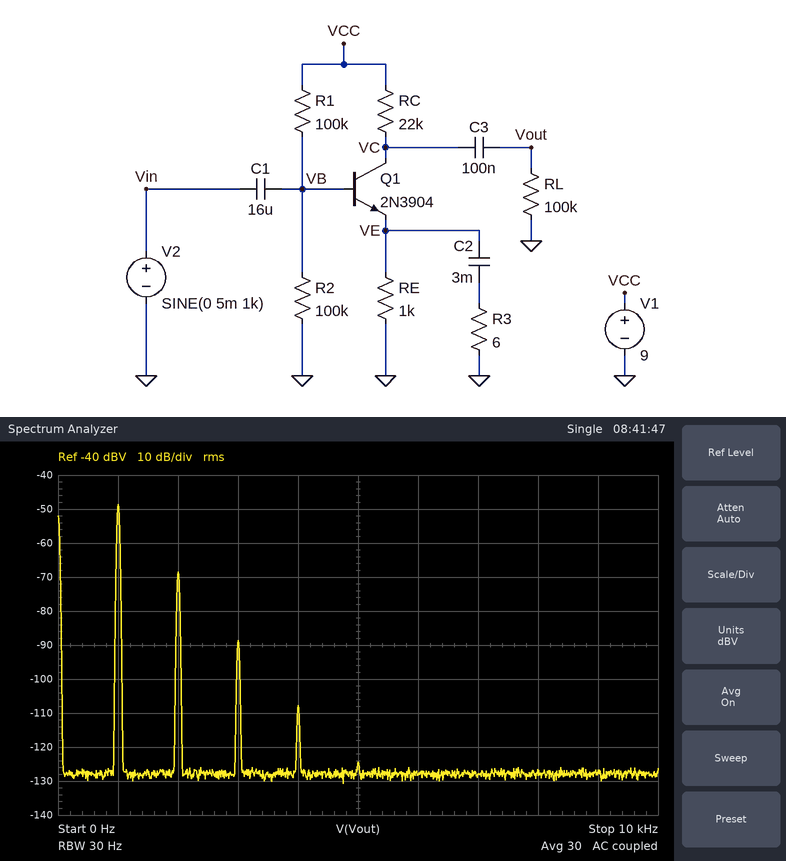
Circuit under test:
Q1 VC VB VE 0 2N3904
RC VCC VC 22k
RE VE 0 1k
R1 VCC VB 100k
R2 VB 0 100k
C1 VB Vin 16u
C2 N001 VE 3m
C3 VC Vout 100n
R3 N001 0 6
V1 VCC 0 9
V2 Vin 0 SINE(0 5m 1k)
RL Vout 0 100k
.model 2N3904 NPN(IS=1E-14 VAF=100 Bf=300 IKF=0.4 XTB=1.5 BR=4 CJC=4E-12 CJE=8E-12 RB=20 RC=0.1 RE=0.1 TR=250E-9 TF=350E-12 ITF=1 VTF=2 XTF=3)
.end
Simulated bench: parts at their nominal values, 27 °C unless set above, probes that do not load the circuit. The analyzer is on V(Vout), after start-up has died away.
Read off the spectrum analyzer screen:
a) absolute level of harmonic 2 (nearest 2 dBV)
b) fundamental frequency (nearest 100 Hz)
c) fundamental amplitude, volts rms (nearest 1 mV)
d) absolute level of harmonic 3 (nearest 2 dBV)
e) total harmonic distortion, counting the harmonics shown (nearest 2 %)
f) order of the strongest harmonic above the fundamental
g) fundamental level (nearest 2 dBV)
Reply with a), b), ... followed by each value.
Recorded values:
a) -68 dBV
b) 1.0 kHz
c) 4 mV
d) -88 dBV
e) 10 %
f) 2
g) -48 dBV
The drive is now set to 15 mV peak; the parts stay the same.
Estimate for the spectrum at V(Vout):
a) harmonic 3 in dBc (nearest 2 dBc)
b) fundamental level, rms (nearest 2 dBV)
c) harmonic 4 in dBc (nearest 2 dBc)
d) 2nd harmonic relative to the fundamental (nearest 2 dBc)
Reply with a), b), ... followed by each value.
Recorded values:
a) -14 dBc
b) -34 dBV
c) -20 dBc
d) -8 dBc
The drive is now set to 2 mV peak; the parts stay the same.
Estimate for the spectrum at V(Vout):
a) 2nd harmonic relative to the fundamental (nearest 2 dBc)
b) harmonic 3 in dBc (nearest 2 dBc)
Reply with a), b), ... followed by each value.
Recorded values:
a) -28 dBc
b) -56 dBc
